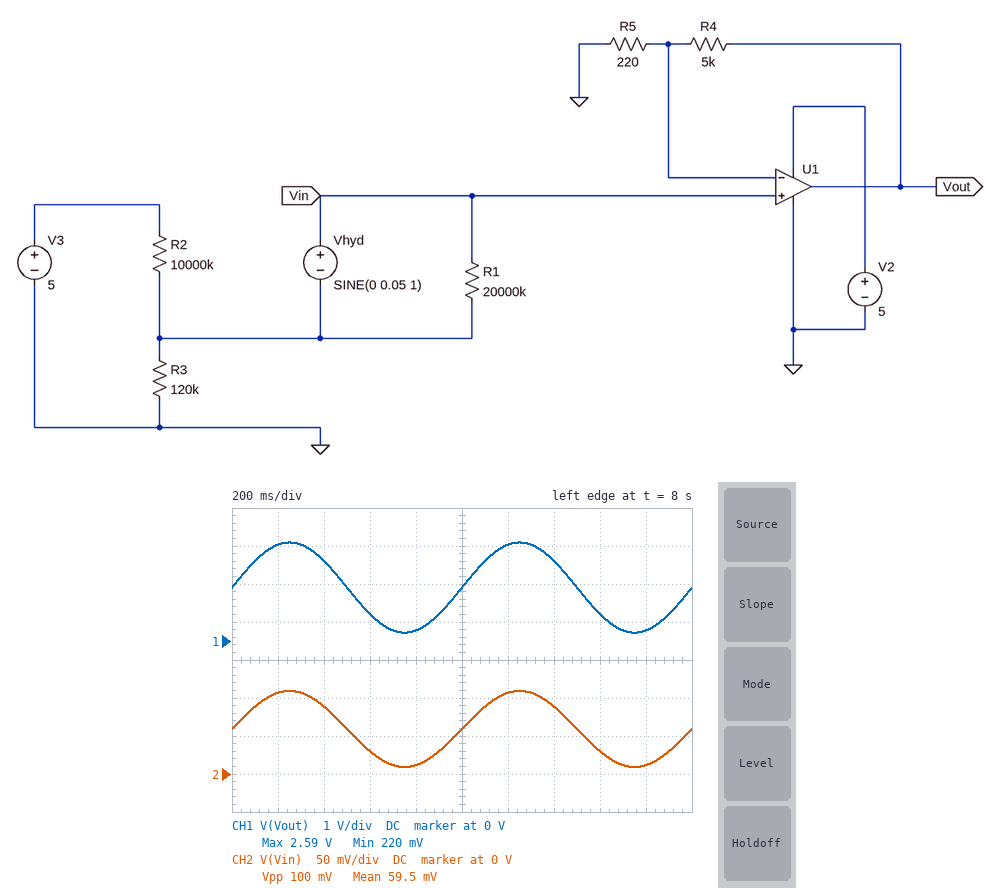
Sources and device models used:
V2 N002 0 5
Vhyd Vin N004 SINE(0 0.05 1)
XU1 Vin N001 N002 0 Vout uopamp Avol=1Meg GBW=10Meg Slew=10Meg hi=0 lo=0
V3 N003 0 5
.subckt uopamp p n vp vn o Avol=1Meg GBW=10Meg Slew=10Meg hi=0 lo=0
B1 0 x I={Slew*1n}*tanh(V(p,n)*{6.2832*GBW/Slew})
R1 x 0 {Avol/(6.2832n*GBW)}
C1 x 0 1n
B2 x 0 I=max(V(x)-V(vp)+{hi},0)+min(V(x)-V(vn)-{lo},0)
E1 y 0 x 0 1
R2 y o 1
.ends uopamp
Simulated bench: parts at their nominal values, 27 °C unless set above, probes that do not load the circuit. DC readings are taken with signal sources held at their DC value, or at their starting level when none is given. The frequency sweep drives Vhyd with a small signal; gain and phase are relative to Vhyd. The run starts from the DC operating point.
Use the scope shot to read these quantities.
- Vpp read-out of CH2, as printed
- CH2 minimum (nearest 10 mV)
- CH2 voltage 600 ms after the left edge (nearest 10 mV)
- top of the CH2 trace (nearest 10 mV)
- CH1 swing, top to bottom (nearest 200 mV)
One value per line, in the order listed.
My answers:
100 mV
10 mV
30 mV
110 mV
2.4 V
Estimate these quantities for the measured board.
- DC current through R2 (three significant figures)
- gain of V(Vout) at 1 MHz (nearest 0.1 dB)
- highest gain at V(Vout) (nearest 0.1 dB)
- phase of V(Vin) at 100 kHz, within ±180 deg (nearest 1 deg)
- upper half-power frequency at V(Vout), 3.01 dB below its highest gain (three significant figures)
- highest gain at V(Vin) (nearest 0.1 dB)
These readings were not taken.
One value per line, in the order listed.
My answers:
494 nA
19.3 dB
27.5 dB
0 deg
421 kHz
0 dB
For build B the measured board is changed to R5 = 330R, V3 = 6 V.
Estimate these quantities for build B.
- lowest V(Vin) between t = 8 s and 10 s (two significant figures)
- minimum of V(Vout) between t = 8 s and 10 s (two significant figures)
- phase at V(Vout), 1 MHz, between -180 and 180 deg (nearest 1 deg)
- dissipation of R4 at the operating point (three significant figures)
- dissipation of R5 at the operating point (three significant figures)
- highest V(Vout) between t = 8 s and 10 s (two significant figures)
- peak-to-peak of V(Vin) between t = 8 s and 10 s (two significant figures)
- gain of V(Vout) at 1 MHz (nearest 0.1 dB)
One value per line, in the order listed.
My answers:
21 mV
340 mV
-58 deg
232 µW
15.3 µW
2.0 V
100 mV
18.6 dB
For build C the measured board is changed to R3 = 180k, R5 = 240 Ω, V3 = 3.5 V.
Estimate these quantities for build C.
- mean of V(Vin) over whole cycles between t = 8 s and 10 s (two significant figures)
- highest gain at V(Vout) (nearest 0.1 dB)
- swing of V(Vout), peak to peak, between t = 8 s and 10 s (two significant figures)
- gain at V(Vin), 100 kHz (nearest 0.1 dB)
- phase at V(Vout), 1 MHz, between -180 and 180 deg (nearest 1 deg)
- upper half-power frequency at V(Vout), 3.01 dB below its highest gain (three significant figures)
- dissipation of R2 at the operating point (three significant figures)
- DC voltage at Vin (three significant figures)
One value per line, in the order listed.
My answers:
62 mV
26.8 dB
2.2 V
0 dB
-65 deg
458 kHz
1.18 µW
61.9 mV
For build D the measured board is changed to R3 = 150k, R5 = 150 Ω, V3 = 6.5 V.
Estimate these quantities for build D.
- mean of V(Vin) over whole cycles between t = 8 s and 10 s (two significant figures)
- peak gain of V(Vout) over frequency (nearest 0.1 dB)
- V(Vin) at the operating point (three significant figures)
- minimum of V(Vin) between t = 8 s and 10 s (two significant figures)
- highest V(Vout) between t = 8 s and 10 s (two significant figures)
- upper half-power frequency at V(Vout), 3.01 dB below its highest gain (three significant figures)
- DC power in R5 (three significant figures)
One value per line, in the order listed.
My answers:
96 mV
30.7 dB
96.1 mV
46 mV
5.0 V
291 kHz
61.5 µW
